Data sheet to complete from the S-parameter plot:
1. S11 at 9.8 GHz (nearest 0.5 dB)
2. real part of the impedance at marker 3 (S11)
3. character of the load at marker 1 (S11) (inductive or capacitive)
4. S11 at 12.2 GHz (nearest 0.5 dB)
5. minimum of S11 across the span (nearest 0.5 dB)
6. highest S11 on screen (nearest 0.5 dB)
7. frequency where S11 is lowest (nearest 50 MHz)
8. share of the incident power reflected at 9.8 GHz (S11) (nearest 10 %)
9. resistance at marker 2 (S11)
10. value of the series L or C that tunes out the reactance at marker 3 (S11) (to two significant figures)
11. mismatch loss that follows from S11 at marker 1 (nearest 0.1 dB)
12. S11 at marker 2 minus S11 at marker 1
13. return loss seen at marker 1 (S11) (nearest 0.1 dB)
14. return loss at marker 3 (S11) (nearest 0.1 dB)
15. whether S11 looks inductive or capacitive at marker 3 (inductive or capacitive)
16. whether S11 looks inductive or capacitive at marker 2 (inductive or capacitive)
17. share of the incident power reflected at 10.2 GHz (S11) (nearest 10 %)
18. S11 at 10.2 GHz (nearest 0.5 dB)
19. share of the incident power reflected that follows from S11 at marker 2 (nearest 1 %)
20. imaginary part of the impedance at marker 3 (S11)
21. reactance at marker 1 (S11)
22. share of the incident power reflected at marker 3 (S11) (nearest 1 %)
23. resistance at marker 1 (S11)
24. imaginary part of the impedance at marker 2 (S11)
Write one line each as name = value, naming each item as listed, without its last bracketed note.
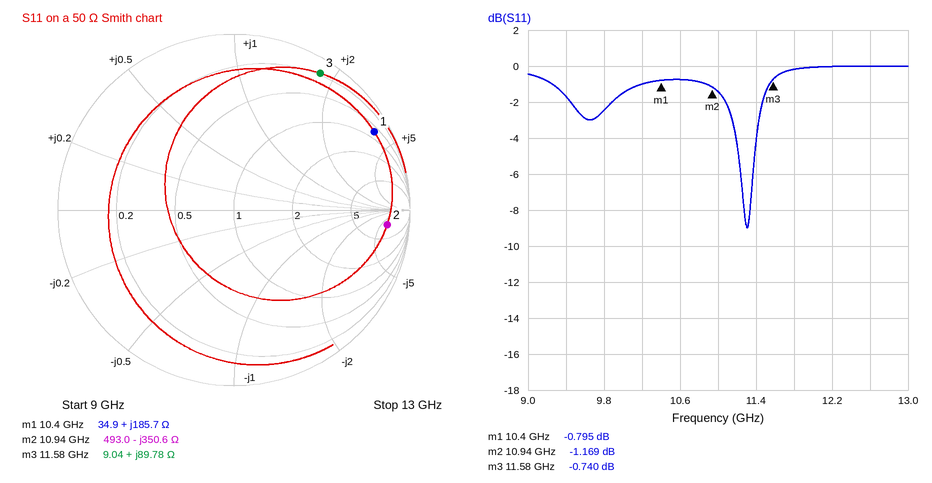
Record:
S11 at 9.8 GHz = -2.5 dB
real part of the impedance at marker 3 = 9.04 Ω
character of the load at marker 1 (S11) = inductive
S11 at 12.2 GHz = 0.0 dB
minimum of S11 across the span = -9.0 dB
highest S11 on screen = 0.0 dB
frequency where S11 is lowest = 11.30 GHz
share of the incident power reflected at 9.8 GHz (S11) = 60 %
resistance at marker 2 = 493.0 Ω
value of the series L or C that tunes out the reactance at marker 3 (S11) = 150 fF
mismatch loss that follows from S11 at marker 1 = 7.8 dB
S11 at marker 2 minus S11 at marker 1 = -0.374 dB
return loss seen at marker 1 (S11) = 0.8 dB
return loss at marker 3 (S11) = 0.7 dB
whether S11 looks inductive or capacitive at marker 3 = inductive
whether S11 looks inductive or capacitive at marker 2 = capacitive
share of the incident power reflected at 10.2 GHz (S11) = 80 %
S11 at 10.2 GHz = -1.0 dB
share of the incident power reflected that follows from S11 at marker 2 = 76 %
imaginary part of the impedance at marker 3 = +89.78 Ω
reactance at marker 1 = +185.7 Ω
share of the incident power reflected at marker 3 (S11) = 84 %
resistance at marker 1 = 34.9 Ω
imaginary part of the impedance at marker 2 = -350.6 Ω
